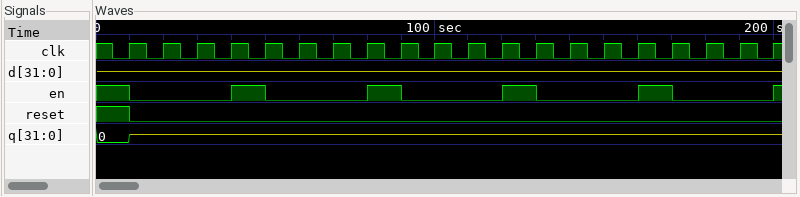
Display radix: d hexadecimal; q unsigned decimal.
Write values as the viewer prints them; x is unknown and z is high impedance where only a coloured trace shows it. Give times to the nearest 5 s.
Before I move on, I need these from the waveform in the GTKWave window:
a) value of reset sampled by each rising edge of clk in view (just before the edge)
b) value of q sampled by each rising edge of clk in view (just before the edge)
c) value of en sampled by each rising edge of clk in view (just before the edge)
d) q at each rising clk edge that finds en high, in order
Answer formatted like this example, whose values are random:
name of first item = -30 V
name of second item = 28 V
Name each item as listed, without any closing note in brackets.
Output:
value of reset sampled by each rising edge of clk in view = 1 0 0 0 0 0 0 0 0 0 0 0 0 0 0 0 0 0 0 0
value of q sampled by each rising edge of clk in view = 0, z, z, z, z, z, z, z, z, z, z, z, z, z, z, z, z, z, z, z
value of en sampled by each rising edge of clk in view = 1 0 0 0 1 0 0 0 1 0 0 0 1 0 0 0 1 0 0 0
q at each rising clk edge that finds en high, in order = 0, z, z, z, z
